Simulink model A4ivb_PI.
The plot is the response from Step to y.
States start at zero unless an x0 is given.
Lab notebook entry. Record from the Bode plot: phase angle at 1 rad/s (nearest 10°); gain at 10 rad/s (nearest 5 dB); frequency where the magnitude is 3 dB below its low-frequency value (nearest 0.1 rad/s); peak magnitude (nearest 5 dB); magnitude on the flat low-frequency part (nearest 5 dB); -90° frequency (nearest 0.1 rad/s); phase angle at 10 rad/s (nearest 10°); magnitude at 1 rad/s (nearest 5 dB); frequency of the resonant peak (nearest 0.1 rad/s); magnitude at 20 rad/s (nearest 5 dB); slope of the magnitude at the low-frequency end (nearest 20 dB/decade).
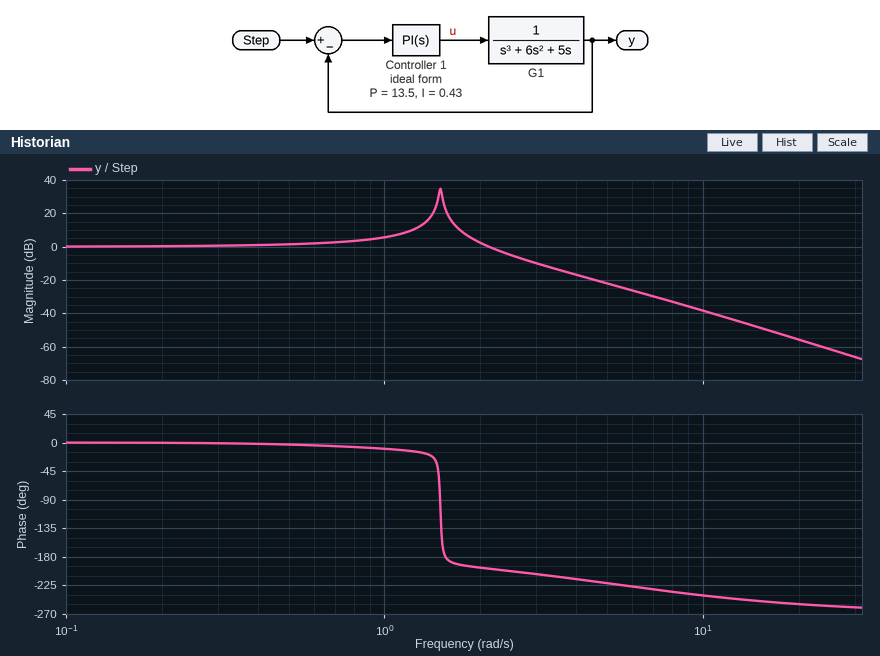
-10°
-40 dB
2.3 rad/s
35 dB
0 dB
1.5 rad/s
-240°
5 dB
1.5 rad/s
-55 dB
0 dB/decade
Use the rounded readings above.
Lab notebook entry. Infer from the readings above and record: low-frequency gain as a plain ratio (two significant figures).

1.0
